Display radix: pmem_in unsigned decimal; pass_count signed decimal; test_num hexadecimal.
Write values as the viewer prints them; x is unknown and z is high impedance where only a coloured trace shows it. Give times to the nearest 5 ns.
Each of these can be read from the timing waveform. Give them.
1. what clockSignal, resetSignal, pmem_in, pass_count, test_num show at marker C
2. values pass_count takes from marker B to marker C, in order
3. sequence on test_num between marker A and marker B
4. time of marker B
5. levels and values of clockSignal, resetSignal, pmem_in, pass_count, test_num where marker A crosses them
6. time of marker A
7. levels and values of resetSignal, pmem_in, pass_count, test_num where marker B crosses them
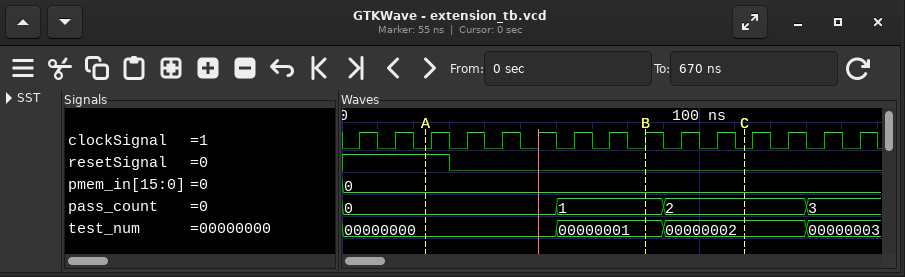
clockSignal=0, resetSignal=0, pmem_in=0, pass_count=2, test_num=00000002
1, 2
00000000, 00000001
85 ns
clockSignal=0, resetSignal=1, pmem_in=0, pass_count=0, test_num=00000000
25 ns
resetSignal=0, pmem_in=0, pass_count=1, test_num=00000001
